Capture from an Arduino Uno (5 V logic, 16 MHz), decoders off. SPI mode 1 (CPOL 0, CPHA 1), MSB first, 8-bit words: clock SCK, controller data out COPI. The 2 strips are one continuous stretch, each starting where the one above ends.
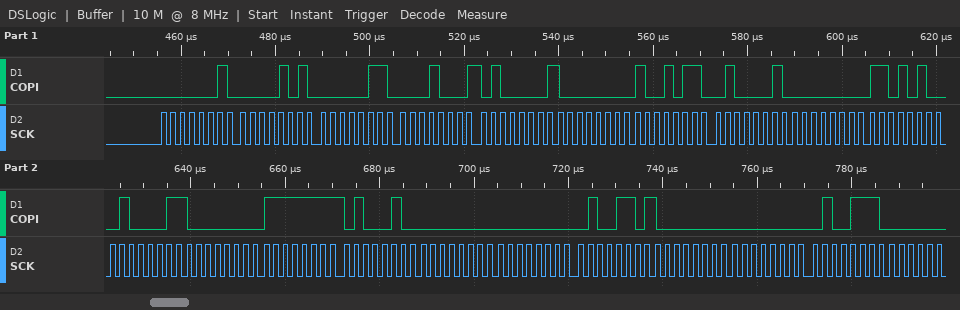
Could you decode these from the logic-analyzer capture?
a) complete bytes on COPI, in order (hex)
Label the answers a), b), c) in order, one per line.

a) 02 0A 06 11 41 00 96 42 00 D4 43 00 FF 44 00 00 4D 00 00 4E
